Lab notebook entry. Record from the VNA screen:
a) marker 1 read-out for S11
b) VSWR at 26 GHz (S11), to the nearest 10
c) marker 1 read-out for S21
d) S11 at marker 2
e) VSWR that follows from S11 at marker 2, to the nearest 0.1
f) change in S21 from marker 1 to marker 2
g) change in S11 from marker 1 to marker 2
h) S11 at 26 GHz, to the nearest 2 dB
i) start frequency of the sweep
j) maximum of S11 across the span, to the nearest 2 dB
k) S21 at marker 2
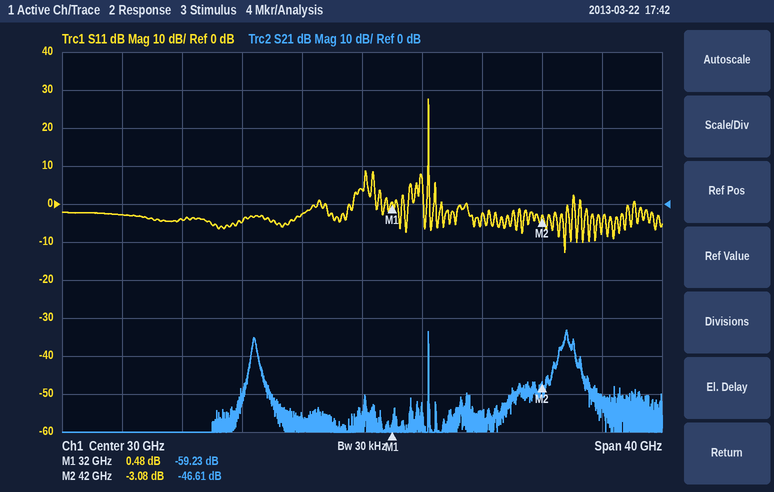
0.48 dB
10
-59.23 dB
-3.08 dB
5.7
12.62 dB
-3.56 dB
-2 dB
10 GHz
28 dB
-46.61 dB
